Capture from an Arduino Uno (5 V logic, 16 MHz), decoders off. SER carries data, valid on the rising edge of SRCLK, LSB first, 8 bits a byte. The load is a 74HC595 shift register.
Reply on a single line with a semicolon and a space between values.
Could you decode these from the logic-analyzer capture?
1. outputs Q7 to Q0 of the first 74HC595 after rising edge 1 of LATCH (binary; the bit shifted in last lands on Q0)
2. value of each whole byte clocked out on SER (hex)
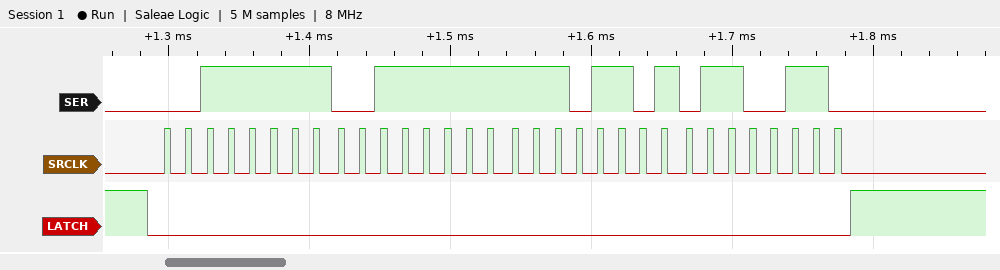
01100110; 0xFC 0xFC 0xB7 0x66
